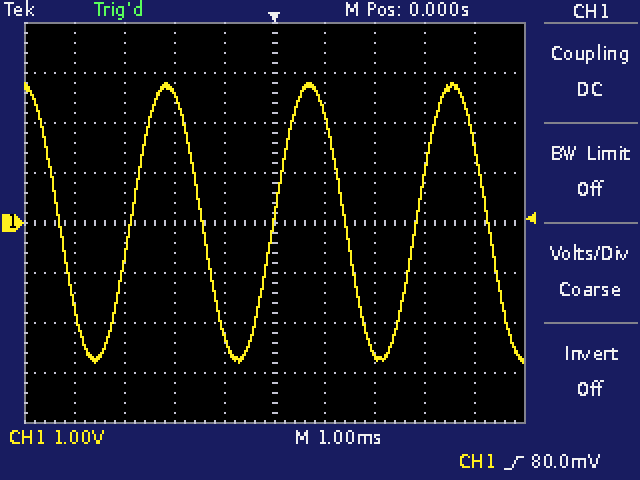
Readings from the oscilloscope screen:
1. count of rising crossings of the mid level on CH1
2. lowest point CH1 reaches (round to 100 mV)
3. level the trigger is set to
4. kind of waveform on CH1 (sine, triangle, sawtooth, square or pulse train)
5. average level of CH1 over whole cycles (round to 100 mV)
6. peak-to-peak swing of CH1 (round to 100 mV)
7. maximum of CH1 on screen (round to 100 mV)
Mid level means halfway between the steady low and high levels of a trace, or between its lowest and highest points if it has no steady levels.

3
-2.8 V
80.0 mV
sine
0.0 V
5.6 V
2.8 V
